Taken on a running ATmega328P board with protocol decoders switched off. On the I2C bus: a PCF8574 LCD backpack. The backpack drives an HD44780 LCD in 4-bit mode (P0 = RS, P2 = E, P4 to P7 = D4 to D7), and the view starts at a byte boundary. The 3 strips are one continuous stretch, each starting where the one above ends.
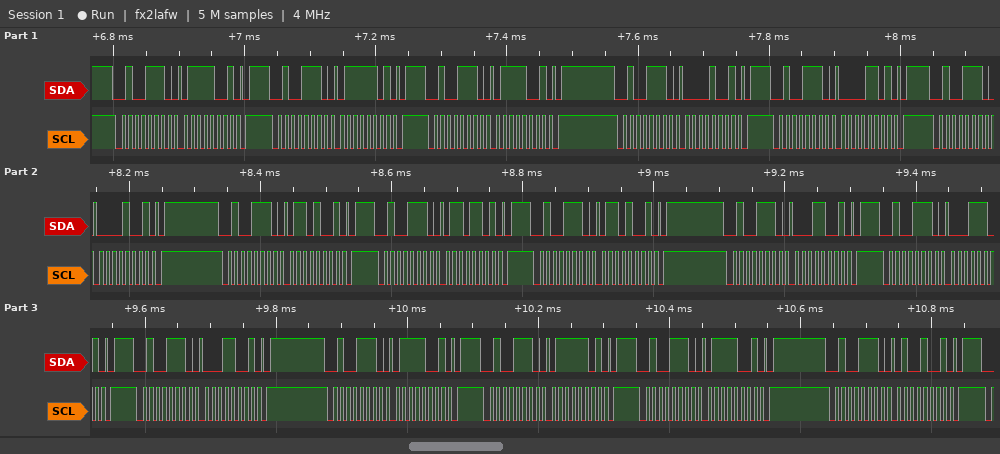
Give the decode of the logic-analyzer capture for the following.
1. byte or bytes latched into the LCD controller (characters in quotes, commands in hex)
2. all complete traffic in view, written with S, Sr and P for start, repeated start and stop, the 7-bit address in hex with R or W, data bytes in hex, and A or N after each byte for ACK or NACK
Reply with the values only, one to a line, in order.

'p' 'a'
S 27W A 79 A P S 27W A 7D A P S 27W A 79 A P S 27W A 09 A P S 27W A 0D A P S 27W A 09 A P S 27W A 69 A P S 27W A 6D A P S 27W A 69 A P S 27W A 19 A P S 27W A 1D A P S 27W A 19 A P S 27W A 79 A P S 27W A 7D A P S 27W A 79 A P S 27W A 49 A P
